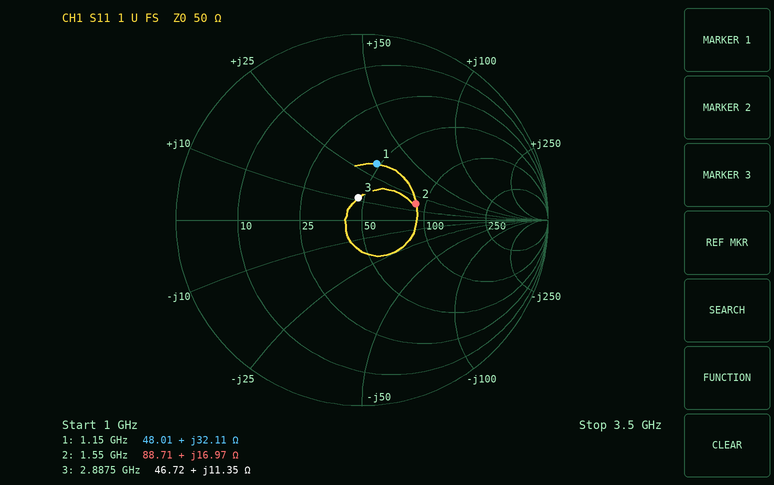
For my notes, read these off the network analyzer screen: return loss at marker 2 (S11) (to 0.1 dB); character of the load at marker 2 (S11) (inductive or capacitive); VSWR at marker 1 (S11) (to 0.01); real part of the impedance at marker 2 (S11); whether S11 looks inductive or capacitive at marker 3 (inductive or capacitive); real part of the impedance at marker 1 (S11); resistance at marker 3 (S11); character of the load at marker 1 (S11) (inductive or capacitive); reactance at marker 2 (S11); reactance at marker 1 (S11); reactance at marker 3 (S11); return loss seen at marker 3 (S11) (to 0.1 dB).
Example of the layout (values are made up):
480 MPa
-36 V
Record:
10.4 dB
inductive
1.91
88.71 Ω
inductive
48.01 Ω
46.72 Ω
inductive
+16.97 Ω
+32.11 Ω
+11.35 Ω
18.3 dB
